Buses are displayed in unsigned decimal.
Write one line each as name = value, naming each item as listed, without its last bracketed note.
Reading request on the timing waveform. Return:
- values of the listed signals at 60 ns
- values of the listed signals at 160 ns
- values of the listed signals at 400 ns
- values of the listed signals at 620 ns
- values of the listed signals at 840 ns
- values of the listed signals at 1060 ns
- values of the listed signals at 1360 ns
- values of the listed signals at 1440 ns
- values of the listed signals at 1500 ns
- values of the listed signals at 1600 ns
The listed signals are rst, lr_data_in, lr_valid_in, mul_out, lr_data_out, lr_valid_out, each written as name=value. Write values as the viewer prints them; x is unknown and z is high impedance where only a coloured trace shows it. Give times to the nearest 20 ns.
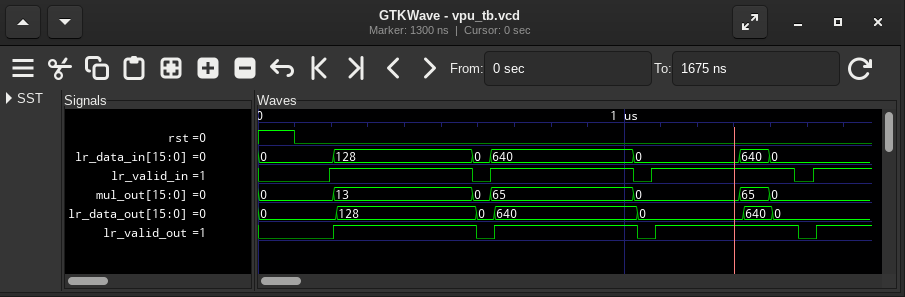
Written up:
values of the listed signals at 60 ns = rst=1, lr_data_in=0, lr_valid_in=0, mul_out=0, lr_data_out=0, lr_valid_out=0
values of the listed signals at 160 ns = rst=0, lr_data_in=0, lr_valid_in=0, mul_out=0, lr_data_out=0, lr_valid_out=0
values of the listed signals at 400 ns = rst=0, lr_data_in=128, lr_valid_in=1, mul_out=13, lr_data_out=128, lr_valid_out=1
values of the listed signals at 620 ns = rst=0, lr_data_in=0, lr_valid_in=0, mul_out=0, lr_data_out=0, lr_valid_out=0
values of the listed signals at 840 ns = rst=0, lr_data_in=640, lr_valid_in=1, mul_out=65, lr_data_out=640, lr_valid_out=1
values of the listed signals at 1060 ns = rst=0, lr_data_in=0, lr_valid_in=0, mul_out=0, lr_data_out=0, lr_valid_out=0
values of the listed signals at 1360 ns = rst=0, lr_data_in=640, lr_valid_in=1, mul_out=65, lr_data_out=640, lr_valid_out=1
values of the listed signals at 1440 ns = rst=0, lr_data_in=0, lr_valid_in=1, mul_out=0, lr_data_out=0, lr_valid_out=1
values of the listed signals at 1500 ns = rst=0, lr_data_in=0, lr_valid_in=0, mul_out=0, lr_data_out=0, lr_valid_out=0
values of the listed signals at 1600 ns = rst=0, lr_data_in=0, lr_valid_in=1, mul_out=0, lr_data_out=0, lr_valid_out=1
